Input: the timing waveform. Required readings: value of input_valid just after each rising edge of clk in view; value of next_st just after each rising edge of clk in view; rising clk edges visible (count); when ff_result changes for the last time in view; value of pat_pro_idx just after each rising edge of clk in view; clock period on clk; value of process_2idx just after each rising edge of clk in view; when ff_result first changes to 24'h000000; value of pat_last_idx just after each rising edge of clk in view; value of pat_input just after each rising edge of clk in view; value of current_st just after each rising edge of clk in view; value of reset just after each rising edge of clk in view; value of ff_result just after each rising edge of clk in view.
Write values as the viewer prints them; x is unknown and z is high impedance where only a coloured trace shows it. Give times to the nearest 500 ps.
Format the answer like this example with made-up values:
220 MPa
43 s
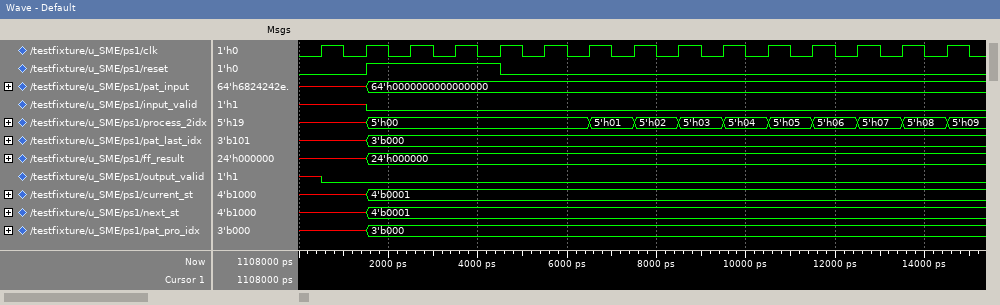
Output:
x 0 0 0 0 0 0 0 0 0 0 0 0 0 0
x, 4'b0001, 4'b0001, 4'b0001, 4'b0001, 4'b0001, 4'b0001, 4'b0001, 4'b0001, 4'b0001, 4'b0001, 4'b0001, 4'b0001, 4'b0001, 4'b0001
15
1500 ps
x, 3'b000, 3'b000, 3'b000, 3'b000, 3'b000, 3'b000, 3'b000, 3'b000, 3'b000, 3'b000, 3'b000, 3'b000, 3'b000, 3'b000
1000 ps
x, 5'h00, 5'h00, 5'h00, 5'h00, 5'h00, 5'h01, 5'h02, 5'h03, 5'h04, 5'h05, 5'h06, 5'h07, 5'h08, 5'h09
1500 ps
x, 3'b000, 3'b000, 3'b000, 3'b000, 3'b000, 3'b000, 3'b000, 3'b000, 3'b000, 3'b000, 3'b000, 3'b000, 3'b000, 3'b000
x, 64'h0000000000000000, 64'h0000000000000000, 64'h0000000000000000, 64'h0000000000000000, 64'h0000000000000000, 64'h0000000000000000, 64'h0000000000000000, 64'h0000000000000000, 64'h0000000000000000, 64'h0000000000000000, 64'h0000000000000000, 64'h0000000000000000, 64'h0000000000000000, 64'h0000000000000000
x, 4'b0001, 4'b0001, 4'b0001, 4'b0001, 4'b0001, 4'b0001, 4'b0001, 4'b0001, 4'b0001, 4'b0001, 4'b0001, 4'b0001, 4'b0001, 4'b0001
0 1 1 1 0 0 0 0 0 0 0 0 0 0 0
x, 24'h000000, 24'h000000, 24'h000000, 24'h000000, 24'h000000, 24'h000000, 24'h000000, 24'h000000, 24'h000000, 24'h000000, 24'h000000, 24'h000000, 24'h000000, 24'h000000
